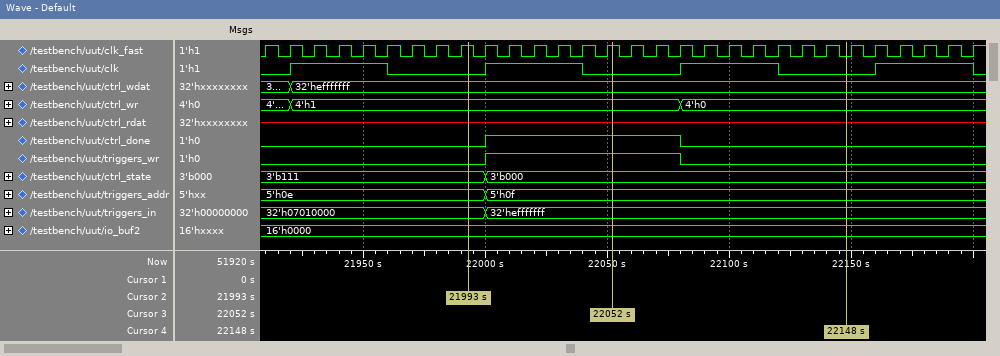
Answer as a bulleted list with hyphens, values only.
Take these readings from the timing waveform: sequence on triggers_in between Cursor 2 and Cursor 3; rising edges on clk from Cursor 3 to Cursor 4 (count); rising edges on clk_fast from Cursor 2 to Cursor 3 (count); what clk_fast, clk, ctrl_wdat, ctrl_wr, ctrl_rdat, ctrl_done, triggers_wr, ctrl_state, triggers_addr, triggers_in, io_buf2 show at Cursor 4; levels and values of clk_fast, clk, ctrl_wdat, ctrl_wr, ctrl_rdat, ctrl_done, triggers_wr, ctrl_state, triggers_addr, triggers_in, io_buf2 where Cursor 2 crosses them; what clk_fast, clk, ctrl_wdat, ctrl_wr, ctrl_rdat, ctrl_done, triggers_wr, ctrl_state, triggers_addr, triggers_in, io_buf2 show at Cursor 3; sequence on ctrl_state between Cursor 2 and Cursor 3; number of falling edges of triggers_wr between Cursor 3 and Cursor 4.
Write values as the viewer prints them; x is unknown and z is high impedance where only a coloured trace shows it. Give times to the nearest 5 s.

- 32'h07010000, 32'hefffffff
- 1
- 6
- clk_fast=0, clk=0, ctrl_wdat=32'hefffffff, ctrl_wr=4'h0, ctrl_rdat=x, ctrl_done=0, triggers_wr=0, ctrl_state=3'b000, triggers_addr=5'h0f, triggers_in=32'hefffffff, io_buf2=16'h0000
- clk_fast=1, clk=0, ctrl_wdat=32'hefffffff, ctrl_wr=4'h1, ctrl_rdat=x, ctrl_done=0, triggers_wr=0, ctrl_state=3'b111, triggers_addr=5'h0e, triggers_in=32'h07010000, io_buf2=16'h0000
- clk_fast=1, clk=0, ctrl_wdat=32'hefffffff, ctrl_wr=4'h1, ctrl_rdat=x, ctrl_done=1, triggers_wr=1, ctrl_state=3'b000, triggers_addr=5'h0f, triggers_in=32'hefffffff, io_buf2=16'h0000
- 3'b111, 3'b000
- 1
